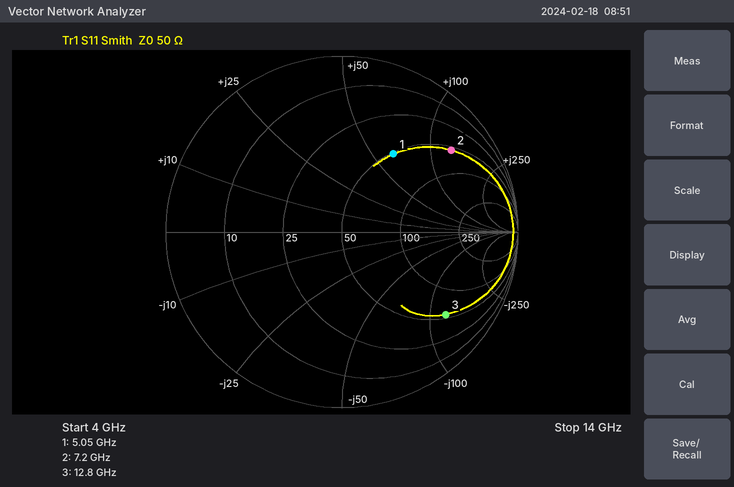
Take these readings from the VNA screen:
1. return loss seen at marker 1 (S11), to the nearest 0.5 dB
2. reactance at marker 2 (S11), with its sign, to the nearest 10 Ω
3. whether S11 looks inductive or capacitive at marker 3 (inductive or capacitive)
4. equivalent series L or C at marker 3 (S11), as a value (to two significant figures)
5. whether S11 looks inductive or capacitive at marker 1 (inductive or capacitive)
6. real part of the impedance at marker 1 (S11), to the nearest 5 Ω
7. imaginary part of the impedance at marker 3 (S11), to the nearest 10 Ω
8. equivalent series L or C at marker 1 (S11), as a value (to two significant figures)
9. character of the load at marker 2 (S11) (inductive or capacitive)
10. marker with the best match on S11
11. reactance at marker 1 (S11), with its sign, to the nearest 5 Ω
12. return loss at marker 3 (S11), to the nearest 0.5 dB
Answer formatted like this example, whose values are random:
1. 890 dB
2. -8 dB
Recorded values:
1. 5.5 dB
2. +130 Ω
3. capacitive
4. 100 fF
5. inductive
6. 50 Ω
7. -120 Ω
8. 2.0 nH
9. inductive
10. marker 1
11. +65 Ω
12. 2.5 dB
